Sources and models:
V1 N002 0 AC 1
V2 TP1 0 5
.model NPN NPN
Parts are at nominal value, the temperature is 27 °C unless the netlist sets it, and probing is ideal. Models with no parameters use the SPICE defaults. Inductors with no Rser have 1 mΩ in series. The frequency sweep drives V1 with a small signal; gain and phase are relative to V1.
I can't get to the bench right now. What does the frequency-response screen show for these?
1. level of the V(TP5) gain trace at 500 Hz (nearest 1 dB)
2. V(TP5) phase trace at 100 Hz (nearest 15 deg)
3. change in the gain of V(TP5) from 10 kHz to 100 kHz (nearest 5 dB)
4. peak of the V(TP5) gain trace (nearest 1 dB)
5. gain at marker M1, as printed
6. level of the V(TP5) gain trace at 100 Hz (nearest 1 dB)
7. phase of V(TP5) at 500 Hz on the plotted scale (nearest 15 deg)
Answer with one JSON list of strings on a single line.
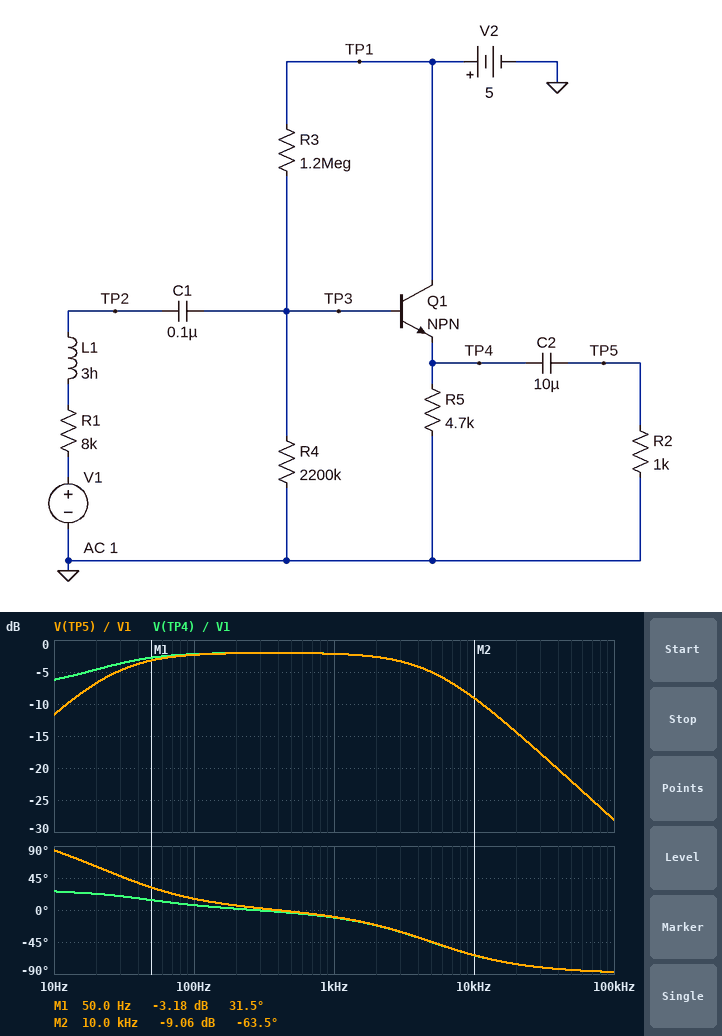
["-2 dB", "15 deg", "-20 dB", "-2 dB", "-3.18 dB", "-2 dB", "0 deg"]
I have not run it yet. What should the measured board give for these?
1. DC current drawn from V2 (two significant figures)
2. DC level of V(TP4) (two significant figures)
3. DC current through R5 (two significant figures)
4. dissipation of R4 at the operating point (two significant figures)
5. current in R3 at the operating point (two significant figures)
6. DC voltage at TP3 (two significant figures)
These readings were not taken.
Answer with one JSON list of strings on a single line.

["200 µA", "950 mV", "200 µA", "1.3 µW", "2.8 µA", "1.7 V"]
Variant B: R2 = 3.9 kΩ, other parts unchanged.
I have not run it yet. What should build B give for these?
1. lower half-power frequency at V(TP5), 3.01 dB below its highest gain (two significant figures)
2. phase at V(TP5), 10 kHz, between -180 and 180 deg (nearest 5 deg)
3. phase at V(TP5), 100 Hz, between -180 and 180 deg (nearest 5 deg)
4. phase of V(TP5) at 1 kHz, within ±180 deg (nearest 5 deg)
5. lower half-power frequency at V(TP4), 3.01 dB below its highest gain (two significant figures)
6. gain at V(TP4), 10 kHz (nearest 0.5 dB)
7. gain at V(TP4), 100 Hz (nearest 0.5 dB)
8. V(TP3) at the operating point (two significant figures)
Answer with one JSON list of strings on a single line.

["11 Hz", "-45 deg", "5 deg", "-5 deg", "9.4 Hz", "-4.0 dB", "-1.0 dB", "1.7 V"]
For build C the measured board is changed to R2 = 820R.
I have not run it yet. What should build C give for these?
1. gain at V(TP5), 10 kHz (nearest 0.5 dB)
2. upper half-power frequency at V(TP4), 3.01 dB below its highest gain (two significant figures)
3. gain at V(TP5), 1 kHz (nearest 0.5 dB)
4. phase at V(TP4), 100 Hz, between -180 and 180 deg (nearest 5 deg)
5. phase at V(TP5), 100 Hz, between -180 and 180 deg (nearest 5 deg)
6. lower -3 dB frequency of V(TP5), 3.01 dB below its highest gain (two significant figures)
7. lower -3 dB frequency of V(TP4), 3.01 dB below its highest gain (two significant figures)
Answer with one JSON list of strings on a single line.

["-10.0 dB", "4.4 kHz", "-2.5 dB", "5 deg", "20 deg", "32 Hz", "18 Hz"]
